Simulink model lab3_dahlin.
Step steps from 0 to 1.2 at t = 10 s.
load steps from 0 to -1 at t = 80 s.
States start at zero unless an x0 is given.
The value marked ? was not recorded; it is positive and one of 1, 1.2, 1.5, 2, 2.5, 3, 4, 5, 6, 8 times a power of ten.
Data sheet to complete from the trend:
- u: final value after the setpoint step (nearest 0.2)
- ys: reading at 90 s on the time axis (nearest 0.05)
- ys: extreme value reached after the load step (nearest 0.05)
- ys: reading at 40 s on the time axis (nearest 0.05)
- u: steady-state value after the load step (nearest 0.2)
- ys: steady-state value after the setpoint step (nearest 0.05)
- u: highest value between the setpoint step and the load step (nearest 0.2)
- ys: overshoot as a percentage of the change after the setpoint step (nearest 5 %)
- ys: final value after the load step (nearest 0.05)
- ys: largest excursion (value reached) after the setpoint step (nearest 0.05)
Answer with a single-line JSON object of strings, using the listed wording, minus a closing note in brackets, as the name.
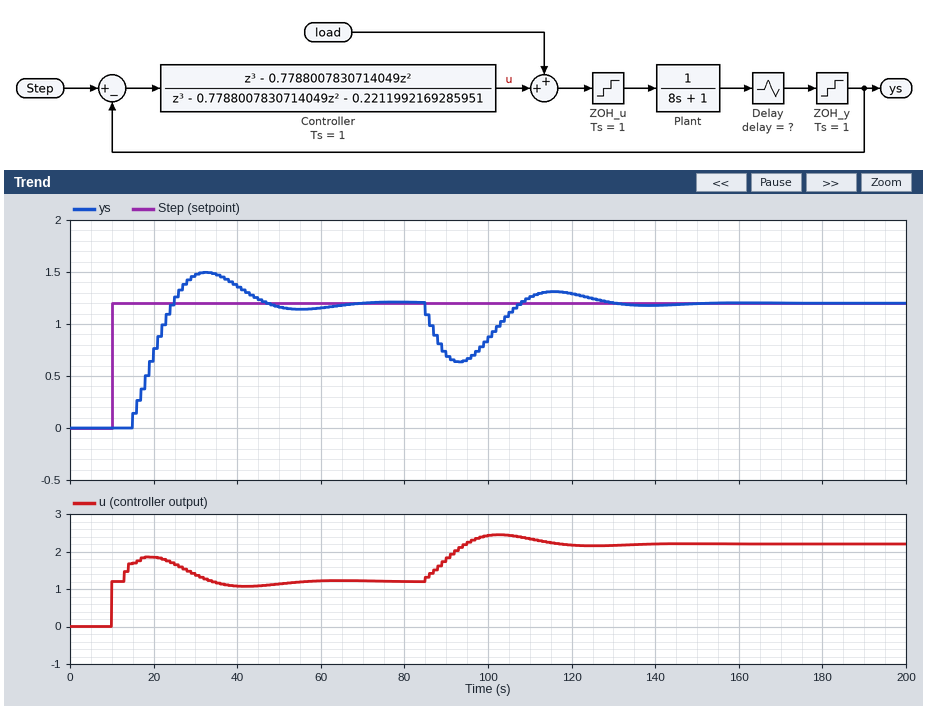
{"u: final value after the setpoint step": "1.2", "ys: reading at 90 s on the time axis": "0.70", "ys: extreme value reached after the load step": "0.65", "ys: reading at 40 s on the time axis": "1.35", "u: steady-state value after the load step": "2.2", "ys: steady-state value after the setpoint step": "1.20", "u: highest value between the setpoint step and the load step": "1.8", "ys: overshoot as a percentage of the change after the setpoint step": "25 %", "ys: final value after the load step": "1.20", "ys: largest excursion (value reached) after the setpoint step": "1.50"}
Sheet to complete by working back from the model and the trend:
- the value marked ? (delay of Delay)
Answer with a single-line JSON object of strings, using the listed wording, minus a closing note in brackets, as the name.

{"the value marked ?": "4"}
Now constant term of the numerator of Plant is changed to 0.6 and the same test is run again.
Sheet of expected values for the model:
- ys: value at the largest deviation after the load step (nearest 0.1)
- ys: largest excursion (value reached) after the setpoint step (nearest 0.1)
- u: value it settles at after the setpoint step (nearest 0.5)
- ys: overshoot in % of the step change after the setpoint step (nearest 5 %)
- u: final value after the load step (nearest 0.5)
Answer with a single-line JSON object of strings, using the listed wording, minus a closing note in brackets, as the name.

{"ys: value at the largest deviation after the load step": "0.8", "ys: largest excursion (value reached) after the setpoint step": "1.3", "u: value it settles at after the setpoint step": "2.0", "ys: overshoot in % of the step change after the setpoint step": "10 %", "u: final value after the load step": "3.0"}
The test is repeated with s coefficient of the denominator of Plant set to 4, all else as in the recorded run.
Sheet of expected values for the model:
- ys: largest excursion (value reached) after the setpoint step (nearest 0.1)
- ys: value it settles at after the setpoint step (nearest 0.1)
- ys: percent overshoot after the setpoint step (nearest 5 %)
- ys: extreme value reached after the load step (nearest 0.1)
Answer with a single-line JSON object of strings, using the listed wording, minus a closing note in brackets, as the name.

{"ys: largest excursion (value reached) after the setpoint step": "1.4", "ys: value it settles at after the setpoint step": "1.2", "ys: percent overshoot after the setpoint step": "15 %", "ys: extreme value reached after the load step": "0.5"}
